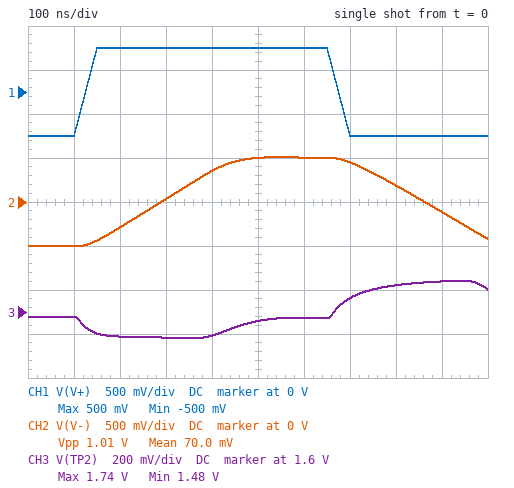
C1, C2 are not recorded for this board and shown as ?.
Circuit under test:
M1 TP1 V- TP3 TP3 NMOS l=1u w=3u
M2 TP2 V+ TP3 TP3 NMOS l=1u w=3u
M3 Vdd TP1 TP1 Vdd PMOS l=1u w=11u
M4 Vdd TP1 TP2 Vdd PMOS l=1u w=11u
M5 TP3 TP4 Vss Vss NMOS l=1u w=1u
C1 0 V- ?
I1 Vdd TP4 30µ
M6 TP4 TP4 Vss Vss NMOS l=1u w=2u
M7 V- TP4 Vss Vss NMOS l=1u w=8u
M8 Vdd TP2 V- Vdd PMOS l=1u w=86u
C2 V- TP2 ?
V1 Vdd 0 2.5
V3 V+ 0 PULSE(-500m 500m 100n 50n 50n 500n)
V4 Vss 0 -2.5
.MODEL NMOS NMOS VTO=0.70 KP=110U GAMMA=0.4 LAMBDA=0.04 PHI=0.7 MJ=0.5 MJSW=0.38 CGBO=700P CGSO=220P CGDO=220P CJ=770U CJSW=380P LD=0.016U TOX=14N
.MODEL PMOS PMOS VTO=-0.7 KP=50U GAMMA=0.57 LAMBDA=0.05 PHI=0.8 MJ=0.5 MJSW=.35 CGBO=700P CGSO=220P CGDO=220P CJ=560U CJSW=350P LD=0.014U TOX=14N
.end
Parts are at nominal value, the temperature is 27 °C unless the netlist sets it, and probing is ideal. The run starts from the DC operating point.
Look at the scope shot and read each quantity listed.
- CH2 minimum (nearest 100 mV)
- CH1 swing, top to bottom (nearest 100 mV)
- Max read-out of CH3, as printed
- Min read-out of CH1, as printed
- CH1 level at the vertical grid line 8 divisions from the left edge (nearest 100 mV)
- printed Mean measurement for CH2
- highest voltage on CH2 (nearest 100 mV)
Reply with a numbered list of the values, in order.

1. -500 mV
2. 1.0 V
3. 1.74 V
4. -500 mV
5. -500 mV
6. 70.0 mV
7. 500 mV
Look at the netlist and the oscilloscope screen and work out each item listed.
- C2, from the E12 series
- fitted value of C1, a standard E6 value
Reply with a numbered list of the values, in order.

1. 4.7 pF
2. 33 pF
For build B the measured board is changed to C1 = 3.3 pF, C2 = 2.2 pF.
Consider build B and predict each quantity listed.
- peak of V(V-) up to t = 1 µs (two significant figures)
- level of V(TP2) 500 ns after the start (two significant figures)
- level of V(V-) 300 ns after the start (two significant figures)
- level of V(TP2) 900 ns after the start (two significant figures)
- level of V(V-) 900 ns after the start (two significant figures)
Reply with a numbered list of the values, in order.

1. 500 mV
2. 1.6 V
3. 490 mV
4. 1.6 V
5. -500 mV
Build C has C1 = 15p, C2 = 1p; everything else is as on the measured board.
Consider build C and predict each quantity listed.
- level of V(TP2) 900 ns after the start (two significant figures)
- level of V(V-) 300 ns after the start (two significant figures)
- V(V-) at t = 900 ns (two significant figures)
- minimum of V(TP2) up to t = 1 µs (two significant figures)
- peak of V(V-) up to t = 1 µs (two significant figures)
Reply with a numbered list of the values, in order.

1. 1.6 V
2. 500 mV
3. -460 mV
4. 1.4 V
5. 550 mV
